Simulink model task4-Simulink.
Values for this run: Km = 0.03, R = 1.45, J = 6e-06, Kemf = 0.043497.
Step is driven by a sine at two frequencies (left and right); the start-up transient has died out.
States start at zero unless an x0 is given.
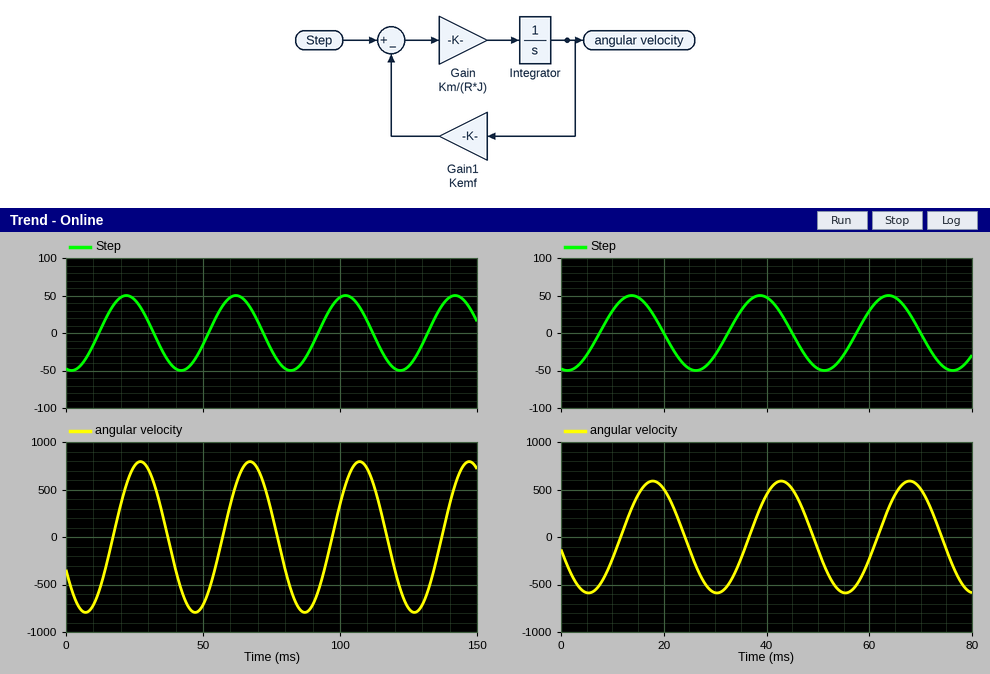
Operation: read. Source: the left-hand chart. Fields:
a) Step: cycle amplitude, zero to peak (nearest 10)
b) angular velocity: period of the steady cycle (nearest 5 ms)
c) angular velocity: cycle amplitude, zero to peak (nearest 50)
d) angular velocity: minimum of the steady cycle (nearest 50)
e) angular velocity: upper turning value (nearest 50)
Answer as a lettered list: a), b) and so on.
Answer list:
a) 50
b) 40 ms
c) 800
d) -800
e) 800
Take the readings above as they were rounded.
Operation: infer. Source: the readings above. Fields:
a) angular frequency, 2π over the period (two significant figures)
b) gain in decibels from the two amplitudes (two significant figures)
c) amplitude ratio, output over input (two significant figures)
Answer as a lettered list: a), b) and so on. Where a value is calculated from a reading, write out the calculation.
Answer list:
a) 2π / 40 = 0.16 rad/ms
b) 20 log10(800 / 50) = 24 dB
c) 800 / 50 = 16
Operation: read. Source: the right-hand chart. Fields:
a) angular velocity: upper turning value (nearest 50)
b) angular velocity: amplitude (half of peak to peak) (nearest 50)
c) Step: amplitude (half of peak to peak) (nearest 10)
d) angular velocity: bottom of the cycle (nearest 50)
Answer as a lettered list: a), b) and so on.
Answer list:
a) 600
b) 600
c) 50
d) -600
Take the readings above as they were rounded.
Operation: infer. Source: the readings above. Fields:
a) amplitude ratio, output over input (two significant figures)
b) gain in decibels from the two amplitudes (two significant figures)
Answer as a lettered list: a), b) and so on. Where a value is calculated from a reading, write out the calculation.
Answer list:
a) 600 / 50 = 12
b) 20 log10(600 / 50) = 22 dB
